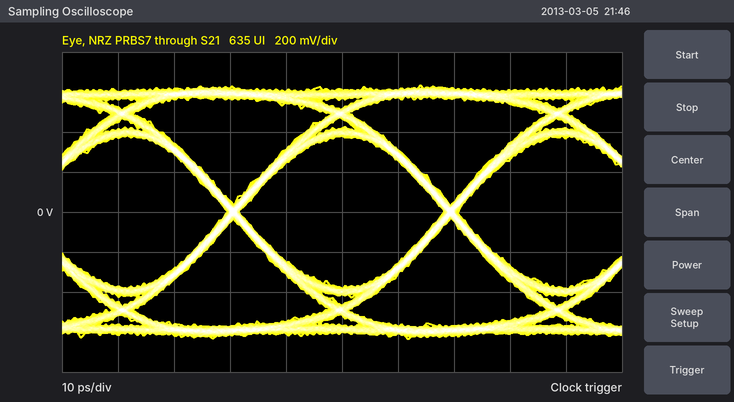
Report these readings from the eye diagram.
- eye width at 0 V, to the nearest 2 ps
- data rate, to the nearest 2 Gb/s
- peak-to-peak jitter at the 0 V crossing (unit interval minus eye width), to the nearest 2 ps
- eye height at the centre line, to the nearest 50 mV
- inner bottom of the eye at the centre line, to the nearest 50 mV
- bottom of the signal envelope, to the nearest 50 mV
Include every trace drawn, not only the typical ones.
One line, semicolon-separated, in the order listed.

36 ps; 26 Gb/s; 2 ps; 750 mV; -400 mV; -650 mV
